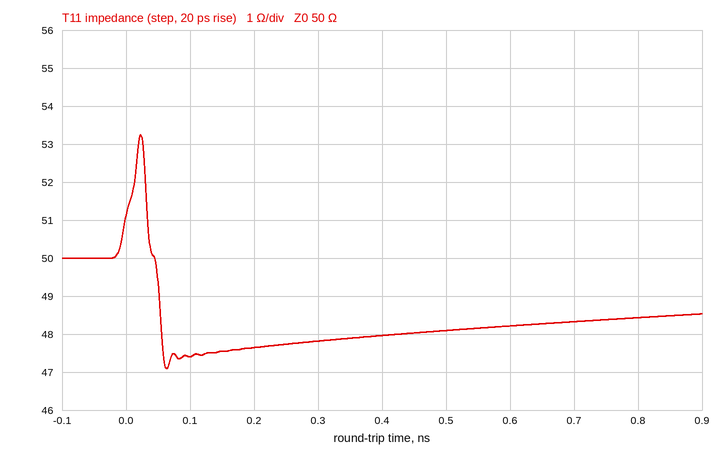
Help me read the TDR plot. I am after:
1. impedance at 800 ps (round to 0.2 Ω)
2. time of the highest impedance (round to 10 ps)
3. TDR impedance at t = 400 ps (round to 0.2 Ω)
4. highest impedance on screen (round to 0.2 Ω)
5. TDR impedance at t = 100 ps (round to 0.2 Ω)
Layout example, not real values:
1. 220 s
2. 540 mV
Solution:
1. 48.4 Ω
2. 20 ps
3. 48.0 Ω
4. 53.2 Ω
5. 47.4 Ω
